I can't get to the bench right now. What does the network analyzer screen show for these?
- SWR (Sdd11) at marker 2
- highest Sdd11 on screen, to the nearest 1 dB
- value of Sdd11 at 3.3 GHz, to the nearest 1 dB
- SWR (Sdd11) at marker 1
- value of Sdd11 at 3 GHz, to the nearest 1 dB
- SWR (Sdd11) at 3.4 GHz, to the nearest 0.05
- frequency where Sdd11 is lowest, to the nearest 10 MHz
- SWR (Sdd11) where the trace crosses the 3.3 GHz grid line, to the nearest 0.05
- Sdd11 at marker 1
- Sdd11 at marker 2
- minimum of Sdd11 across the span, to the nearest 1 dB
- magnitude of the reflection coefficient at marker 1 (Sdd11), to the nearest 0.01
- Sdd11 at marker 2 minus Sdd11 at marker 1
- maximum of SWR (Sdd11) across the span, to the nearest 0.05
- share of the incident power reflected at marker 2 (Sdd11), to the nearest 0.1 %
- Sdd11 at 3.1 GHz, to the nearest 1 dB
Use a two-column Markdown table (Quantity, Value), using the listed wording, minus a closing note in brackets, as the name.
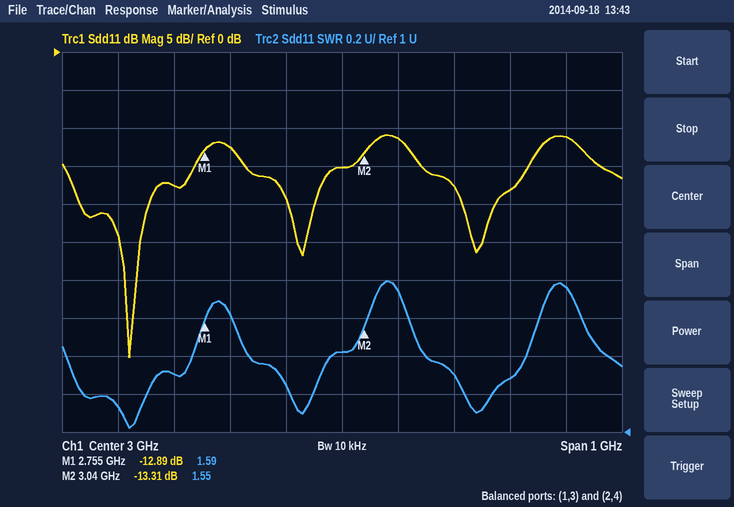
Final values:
| Quantity | Value |
|---|---|
| SWR (Sdd11) at marker 2 | 1.55 |
| highest Sdd11 on screen, to the nearest 1 dB | -11 dB |
| value of Sdd11 at 3.3 GHz, to the nearest 1 dB | -18 dB |
| SWR (Sdd11) at marker 1 | 1.59 |
| value of Sdd11 at 3 GHz, to the nearest 1 dB | -15 dB |
| SWR (Sdd11) at 3.4 GHz, to the nearest 0.05 | 1.75 |
| frequency where Sdd11 is lowest, to the nearest 10 MHz | 2.62 GHz |
| SWR (Sdd11) where the trace crosses the 3.3 GHz grid line, to the nearest 0.05 | 1.30 |
| Sdd11 at marker 1 | -12.89 dB |
| Sdd11 at marker 2 | -13.31 dB |
| minimum of Sdd11 across the span, to the nearest 1 dB | -40 dB |
| magnitude of the reflection coefficient at marker 1 (Sdd11), to the nearest 0.01 | 0.23 |
| Sdd11 at marker 2 minus Sdd11 at marker 1 | -0.42 dB |
| maximum of SWR (Sdd11) across the span, to the nearest 0.05 | 1.80 |
| share of the incident power reflected at marker 2 (Sdd11), to the nearest 0.1 % | 4.7 % |
| Sdd11 at 3.1 GHz, to the nearest 1 dB | -11 dB |
